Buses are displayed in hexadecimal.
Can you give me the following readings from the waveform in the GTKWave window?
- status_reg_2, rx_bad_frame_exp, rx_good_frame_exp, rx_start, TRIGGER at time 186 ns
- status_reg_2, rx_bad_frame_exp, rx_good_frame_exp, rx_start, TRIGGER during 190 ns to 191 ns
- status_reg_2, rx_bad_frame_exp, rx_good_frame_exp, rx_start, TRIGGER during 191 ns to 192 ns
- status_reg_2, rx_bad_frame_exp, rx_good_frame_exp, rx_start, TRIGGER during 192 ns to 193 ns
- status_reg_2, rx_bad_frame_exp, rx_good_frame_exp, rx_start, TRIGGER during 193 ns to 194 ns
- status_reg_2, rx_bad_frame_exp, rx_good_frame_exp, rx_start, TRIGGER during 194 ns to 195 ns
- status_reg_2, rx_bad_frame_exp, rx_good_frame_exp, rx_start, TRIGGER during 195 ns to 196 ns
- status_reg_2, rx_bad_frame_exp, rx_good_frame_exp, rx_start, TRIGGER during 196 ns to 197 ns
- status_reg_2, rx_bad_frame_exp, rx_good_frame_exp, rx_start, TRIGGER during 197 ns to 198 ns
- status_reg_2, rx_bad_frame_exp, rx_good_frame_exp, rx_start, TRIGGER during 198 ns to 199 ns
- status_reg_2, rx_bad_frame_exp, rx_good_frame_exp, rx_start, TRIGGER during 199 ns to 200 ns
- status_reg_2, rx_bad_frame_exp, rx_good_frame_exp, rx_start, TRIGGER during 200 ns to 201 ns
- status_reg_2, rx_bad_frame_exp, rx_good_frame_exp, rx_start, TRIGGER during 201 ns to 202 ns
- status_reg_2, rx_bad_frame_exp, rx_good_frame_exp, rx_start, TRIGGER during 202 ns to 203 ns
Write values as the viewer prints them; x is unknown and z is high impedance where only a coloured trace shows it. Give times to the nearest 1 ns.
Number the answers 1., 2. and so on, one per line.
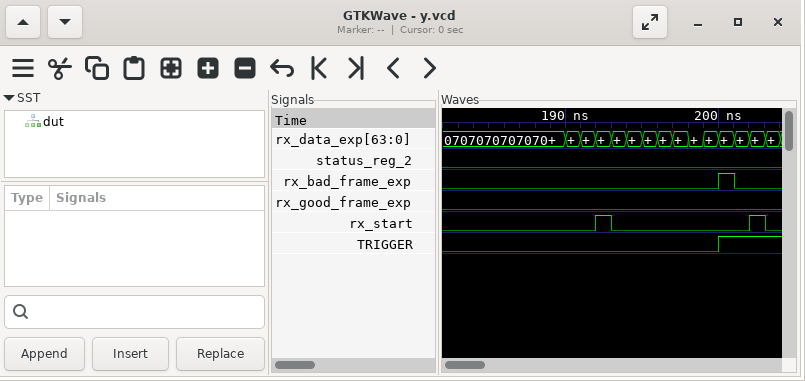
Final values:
1. status_reg_2=0, rx_bad_frame_exp=0, rx_good_frame_exp=0, rx_start=0, TRIGGER=0
2. status_reg_2=0, rx_bad_frame_exp=0, rx_good_frame_exp=0, rx_start=0, TRIGGER=0
3. status_reg_2=0, rx_bad_frame_exp=0, rx_good_frame_exp=0, rx_start=0, TRIGGER=0
4. status_reg_2=0, rx_bad_frame_exp=0, rx_good_frame_exp=0, rx_start=1, TRIGGER=0
5. status_reg_2=0, rx_bad_frame_exp=0, rx_good_frame_exp=0, rx_start=0, TRIGGER=0
6. status_reg_2=0, rx_bad_frame_exp=0, rx_good_frame_exp=0, rx_start=0, TRIGGER=0
7. status_reg_2=0, rx_bad_frame_exp=0, rx_good_frame_exp=0, rx_start=0, TRIGGER=0
8. status_reg_2=0, rx_bad_frame_exp=0, rx_good_frame_exp=0, rx_start=0, TRIGGER=0
9. status_reg_2=0, rx_bad_frame_exp=0, rx_good_frame_exp=0, rx_start=0, TRIGGER=0
10. status_reg_2=0, rx_bad_frame_exp=0, rx_good_frame_exp=0, rx_start=0, TRIGGER=0
11. status_reg_2=0, rx_bad_frame_exp=0, rx_good_frame_exp=0, rx_start=0, TRIGGER=0
12. status_reg_2=0, rx_bad_frame_exp=1, rx_good_frame_exp=0, rx_start=0, TRIGGER=1
13. status_reg_2=0, rx_bad_frame_exp=0, rx_good_frame_exp=0, rx_start=0, TRIGGER=1
14. status_reg_2=0, rx_bad_frame_exp=0, rx_good_frame_exp=0, rx_start=1, TRIGGER=1
